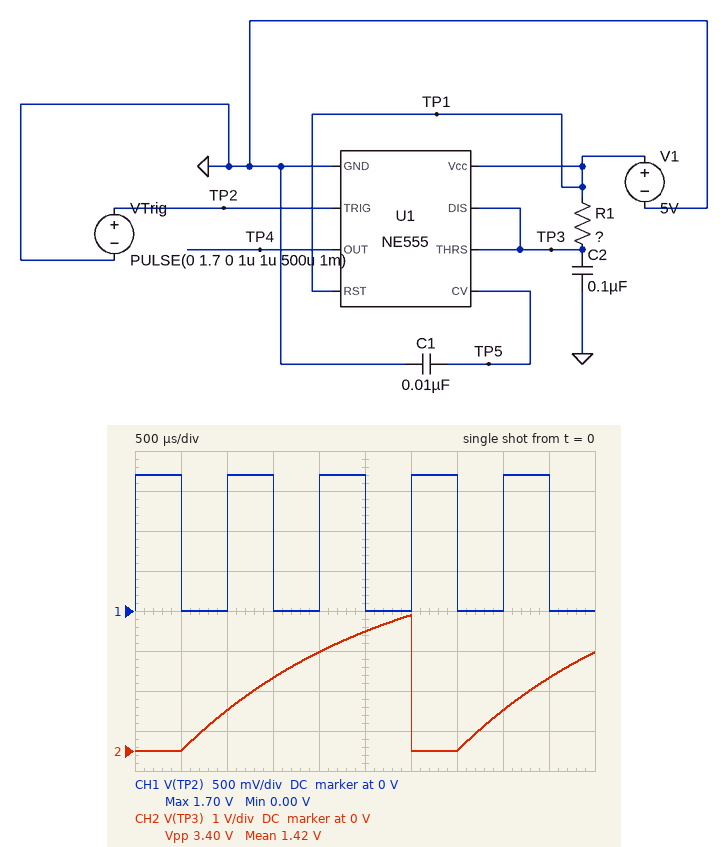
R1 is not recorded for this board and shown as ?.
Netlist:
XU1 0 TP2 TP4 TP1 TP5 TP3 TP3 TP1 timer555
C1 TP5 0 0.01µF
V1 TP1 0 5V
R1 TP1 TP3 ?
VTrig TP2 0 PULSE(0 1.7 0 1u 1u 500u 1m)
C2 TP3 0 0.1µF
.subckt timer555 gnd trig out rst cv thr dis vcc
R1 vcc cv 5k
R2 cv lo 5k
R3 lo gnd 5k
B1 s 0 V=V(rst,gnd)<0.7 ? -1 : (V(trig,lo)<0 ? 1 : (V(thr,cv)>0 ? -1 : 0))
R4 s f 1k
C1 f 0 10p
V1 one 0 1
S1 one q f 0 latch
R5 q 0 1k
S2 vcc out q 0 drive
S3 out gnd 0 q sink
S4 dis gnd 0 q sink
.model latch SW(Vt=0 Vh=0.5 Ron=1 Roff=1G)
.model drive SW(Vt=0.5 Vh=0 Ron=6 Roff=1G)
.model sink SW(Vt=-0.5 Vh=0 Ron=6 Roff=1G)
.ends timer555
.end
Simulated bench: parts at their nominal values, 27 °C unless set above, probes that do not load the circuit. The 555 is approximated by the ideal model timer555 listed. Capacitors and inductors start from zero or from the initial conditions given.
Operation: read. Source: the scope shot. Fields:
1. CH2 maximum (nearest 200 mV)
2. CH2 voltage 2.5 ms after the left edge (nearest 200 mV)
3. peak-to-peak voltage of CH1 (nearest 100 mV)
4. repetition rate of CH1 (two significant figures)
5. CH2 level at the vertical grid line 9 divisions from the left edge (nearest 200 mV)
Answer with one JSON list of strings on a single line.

["3.4 V", "3.0 V", "1.7 V", "1.0 kHz", "1.8 V"]
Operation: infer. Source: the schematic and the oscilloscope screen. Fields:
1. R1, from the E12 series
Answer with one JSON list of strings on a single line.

["22 kΩ"]
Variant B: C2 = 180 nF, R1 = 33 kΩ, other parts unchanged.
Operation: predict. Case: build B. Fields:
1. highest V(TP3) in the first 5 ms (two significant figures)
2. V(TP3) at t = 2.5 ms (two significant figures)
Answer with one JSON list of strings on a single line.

["2.7 V", "1.4 V"]
